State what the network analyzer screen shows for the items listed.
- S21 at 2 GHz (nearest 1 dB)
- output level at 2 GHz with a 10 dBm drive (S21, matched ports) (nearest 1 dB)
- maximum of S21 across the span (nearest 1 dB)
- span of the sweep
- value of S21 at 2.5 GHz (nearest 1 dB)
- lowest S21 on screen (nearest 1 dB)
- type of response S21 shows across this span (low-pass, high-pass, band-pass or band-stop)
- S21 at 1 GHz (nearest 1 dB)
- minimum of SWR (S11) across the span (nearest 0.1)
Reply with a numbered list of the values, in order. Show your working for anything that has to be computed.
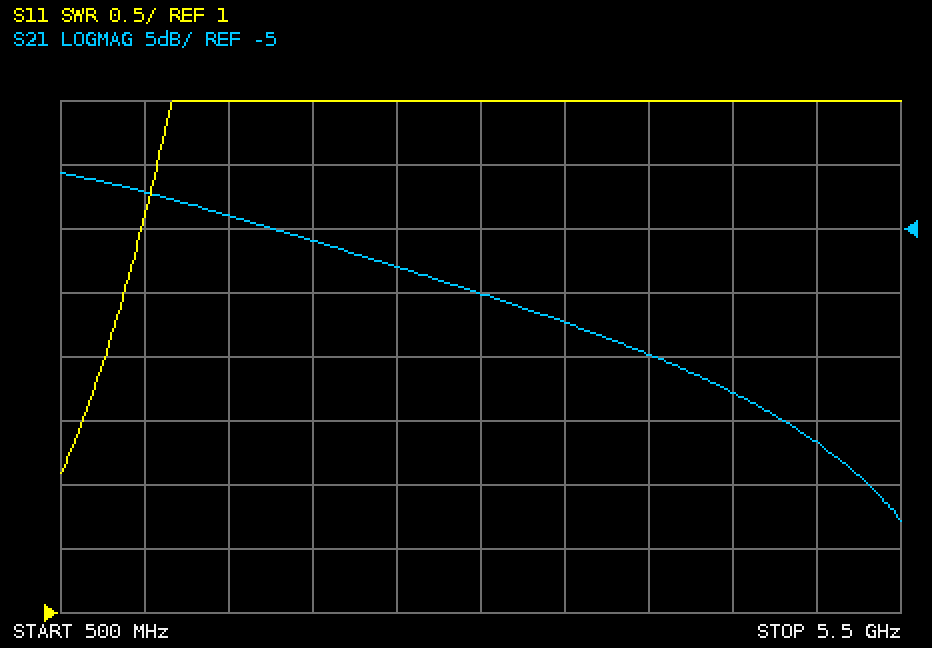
1. -6 dB
2. 10 dBm + (-6 dB) = 4 dBm
3. -1 dB
4. 5 GHz
5. -8 dB
6. -28 dB
7. low-pass
8. -2 dB
9. 2.1
